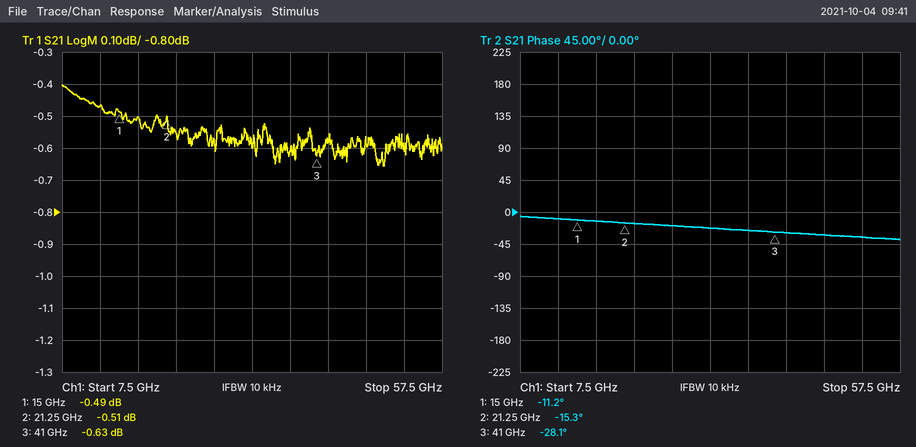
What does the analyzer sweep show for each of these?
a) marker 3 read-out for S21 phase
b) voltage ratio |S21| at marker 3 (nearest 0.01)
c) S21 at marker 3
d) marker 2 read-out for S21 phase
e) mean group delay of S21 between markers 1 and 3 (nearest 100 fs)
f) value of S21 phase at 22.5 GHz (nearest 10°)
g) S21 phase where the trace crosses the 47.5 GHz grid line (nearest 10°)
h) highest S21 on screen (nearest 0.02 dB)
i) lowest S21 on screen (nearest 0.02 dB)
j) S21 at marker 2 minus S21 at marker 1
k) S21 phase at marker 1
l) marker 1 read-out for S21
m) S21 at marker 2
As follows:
-28.1°
0.93
-0.63 dB
-15.3°
1.8 ps
-20°
-30°
-0.40 dB
-0.66 dB
-0.02 dB
-11.2°
-0.49 dB
-0.51 dB
